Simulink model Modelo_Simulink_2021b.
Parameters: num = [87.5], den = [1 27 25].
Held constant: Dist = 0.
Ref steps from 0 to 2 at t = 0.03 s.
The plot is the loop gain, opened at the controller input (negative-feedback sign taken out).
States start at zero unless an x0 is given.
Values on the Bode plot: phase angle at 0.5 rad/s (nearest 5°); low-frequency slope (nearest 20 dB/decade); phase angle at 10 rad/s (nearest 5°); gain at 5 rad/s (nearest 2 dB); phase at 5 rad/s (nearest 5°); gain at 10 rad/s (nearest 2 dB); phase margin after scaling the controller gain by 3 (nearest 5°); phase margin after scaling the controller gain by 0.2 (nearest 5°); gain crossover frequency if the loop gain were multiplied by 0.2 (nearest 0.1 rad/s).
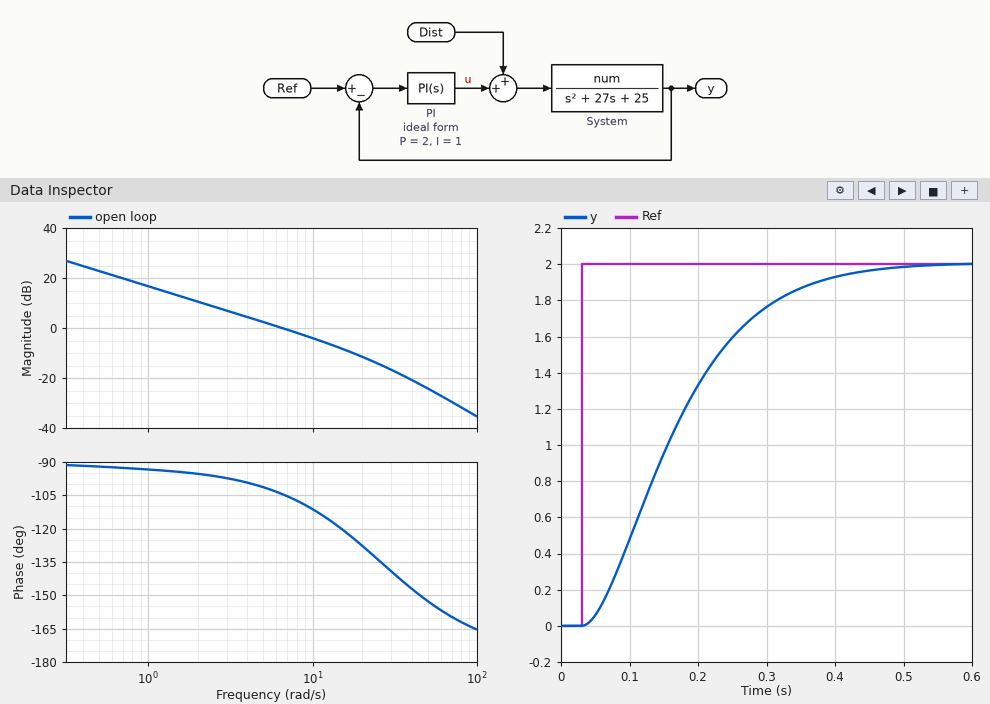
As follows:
-90°
-20 dB/decade
-110°
2 dB
-100°
-4 dB
55°
85°
1.4 rad/s
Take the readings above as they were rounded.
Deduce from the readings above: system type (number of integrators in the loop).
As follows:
1
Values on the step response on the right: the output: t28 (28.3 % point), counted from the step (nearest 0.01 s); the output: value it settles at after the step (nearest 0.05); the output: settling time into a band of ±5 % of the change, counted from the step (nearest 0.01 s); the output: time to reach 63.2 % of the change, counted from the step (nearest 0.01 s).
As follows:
0.08 s
2.00
0.34 s
0.16 s
